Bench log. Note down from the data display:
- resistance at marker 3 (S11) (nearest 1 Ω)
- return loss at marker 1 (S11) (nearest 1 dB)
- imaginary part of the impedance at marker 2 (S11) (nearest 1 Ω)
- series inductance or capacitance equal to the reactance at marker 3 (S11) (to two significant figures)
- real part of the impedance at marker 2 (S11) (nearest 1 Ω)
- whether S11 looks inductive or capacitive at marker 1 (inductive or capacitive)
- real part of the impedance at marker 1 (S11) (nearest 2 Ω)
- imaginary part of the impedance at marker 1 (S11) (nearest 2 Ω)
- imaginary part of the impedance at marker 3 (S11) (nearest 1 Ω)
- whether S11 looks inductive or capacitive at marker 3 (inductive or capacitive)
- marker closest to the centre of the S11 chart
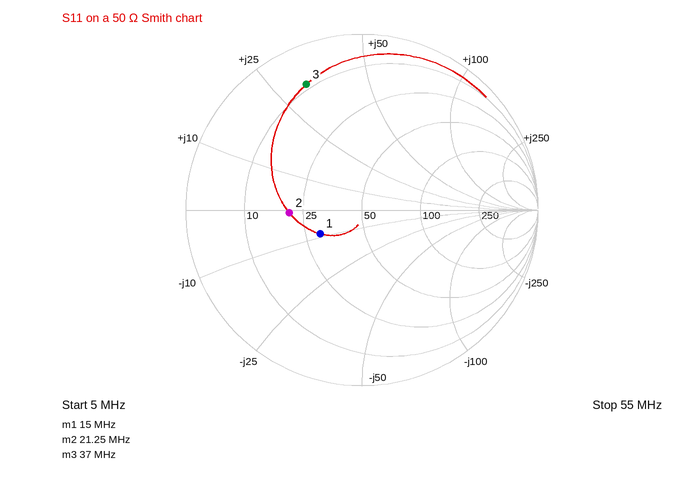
9 Ω
11 dB
-1 Ω
140 nH
21 Ω
capacitive
30 Ω
-8 Ω
+32 Ω
inductive
marker 1
